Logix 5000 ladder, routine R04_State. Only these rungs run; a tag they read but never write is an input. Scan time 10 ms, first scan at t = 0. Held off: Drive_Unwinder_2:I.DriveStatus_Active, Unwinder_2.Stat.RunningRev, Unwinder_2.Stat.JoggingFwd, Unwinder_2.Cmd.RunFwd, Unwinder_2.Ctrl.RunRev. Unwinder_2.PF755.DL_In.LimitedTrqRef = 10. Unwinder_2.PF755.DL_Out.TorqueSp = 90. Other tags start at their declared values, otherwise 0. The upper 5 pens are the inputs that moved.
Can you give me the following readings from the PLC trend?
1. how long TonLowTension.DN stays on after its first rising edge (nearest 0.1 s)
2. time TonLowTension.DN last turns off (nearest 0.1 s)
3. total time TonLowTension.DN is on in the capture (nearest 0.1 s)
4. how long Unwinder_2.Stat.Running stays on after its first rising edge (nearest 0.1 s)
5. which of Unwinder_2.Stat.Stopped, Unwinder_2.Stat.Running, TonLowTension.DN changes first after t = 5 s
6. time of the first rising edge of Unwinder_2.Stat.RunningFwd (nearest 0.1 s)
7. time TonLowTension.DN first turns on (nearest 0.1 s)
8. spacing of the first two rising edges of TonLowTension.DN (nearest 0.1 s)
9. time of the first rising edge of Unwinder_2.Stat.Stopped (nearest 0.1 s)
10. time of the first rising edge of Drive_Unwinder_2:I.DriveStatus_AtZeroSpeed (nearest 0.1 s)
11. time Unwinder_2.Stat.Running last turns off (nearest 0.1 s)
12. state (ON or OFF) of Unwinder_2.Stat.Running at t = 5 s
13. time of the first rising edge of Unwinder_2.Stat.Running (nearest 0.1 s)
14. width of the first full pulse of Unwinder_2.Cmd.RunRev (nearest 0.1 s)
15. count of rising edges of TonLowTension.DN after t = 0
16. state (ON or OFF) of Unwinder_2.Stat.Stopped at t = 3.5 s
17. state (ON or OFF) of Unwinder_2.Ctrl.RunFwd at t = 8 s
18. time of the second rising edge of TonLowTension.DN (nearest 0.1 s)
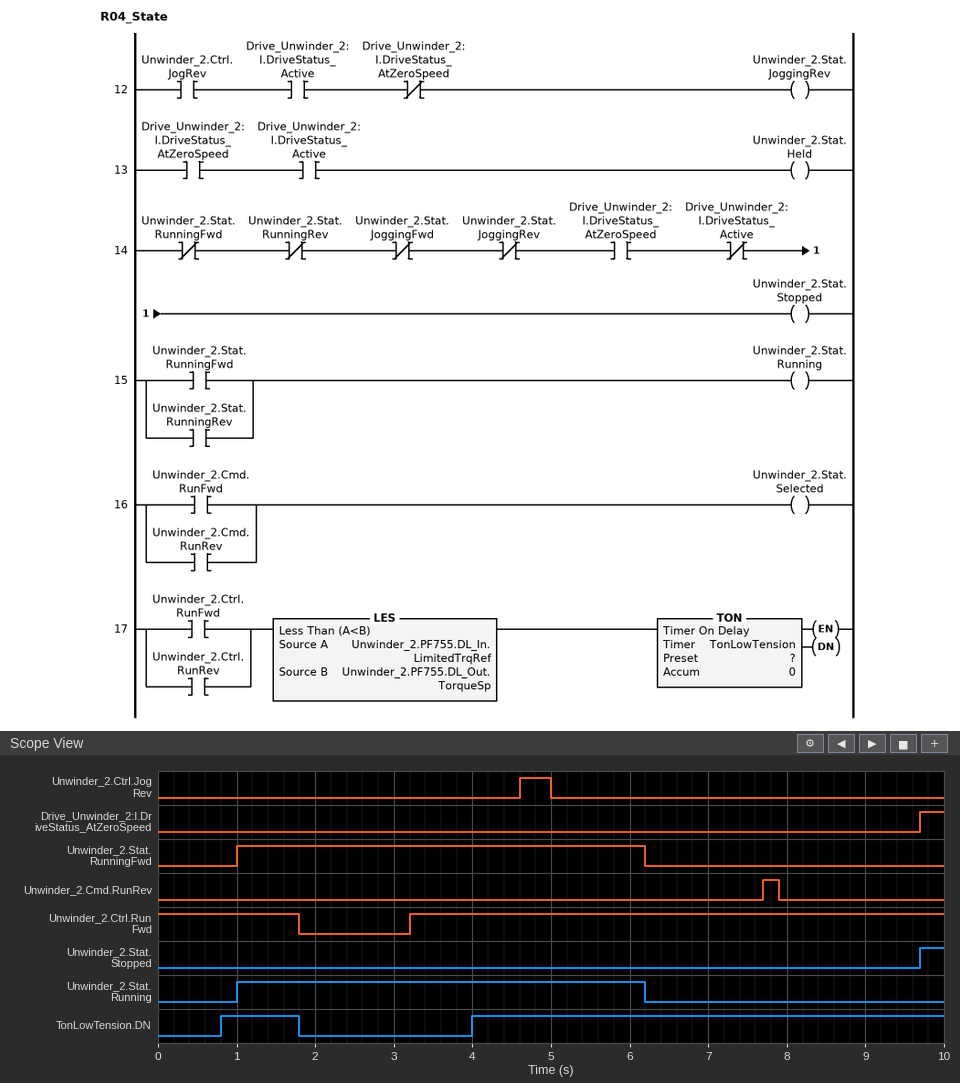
1.0 s
1.8 s
7.0 s
5.2 s
Unwinder_2.Stat.Running
1.0 s
0.8 s
3.2 s
9.7 s
9.7 s
6.2 s
ON
1.0 s
0.2 s
2
OFF
ON
4.0 s
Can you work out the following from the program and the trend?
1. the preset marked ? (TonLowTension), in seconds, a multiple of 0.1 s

0.8 s
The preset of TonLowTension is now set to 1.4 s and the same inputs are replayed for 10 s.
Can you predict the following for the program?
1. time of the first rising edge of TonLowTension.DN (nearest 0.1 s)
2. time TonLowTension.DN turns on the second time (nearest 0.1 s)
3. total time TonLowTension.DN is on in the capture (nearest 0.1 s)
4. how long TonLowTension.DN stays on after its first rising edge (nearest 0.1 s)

1.4 s
4.6 s
5.8 s
0.4 s
